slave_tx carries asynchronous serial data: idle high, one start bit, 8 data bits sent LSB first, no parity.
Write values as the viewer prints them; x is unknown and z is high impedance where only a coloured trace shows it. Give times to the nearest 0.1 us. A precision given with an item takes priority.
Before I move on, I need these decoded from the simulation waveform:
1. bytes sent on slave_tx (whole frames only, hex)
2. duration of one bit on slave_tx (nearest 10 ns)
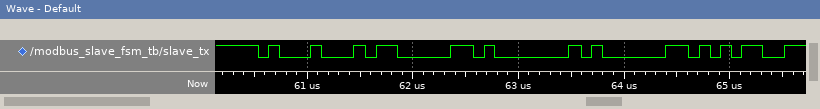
11, 83, 01, 81, 35
100 ns
